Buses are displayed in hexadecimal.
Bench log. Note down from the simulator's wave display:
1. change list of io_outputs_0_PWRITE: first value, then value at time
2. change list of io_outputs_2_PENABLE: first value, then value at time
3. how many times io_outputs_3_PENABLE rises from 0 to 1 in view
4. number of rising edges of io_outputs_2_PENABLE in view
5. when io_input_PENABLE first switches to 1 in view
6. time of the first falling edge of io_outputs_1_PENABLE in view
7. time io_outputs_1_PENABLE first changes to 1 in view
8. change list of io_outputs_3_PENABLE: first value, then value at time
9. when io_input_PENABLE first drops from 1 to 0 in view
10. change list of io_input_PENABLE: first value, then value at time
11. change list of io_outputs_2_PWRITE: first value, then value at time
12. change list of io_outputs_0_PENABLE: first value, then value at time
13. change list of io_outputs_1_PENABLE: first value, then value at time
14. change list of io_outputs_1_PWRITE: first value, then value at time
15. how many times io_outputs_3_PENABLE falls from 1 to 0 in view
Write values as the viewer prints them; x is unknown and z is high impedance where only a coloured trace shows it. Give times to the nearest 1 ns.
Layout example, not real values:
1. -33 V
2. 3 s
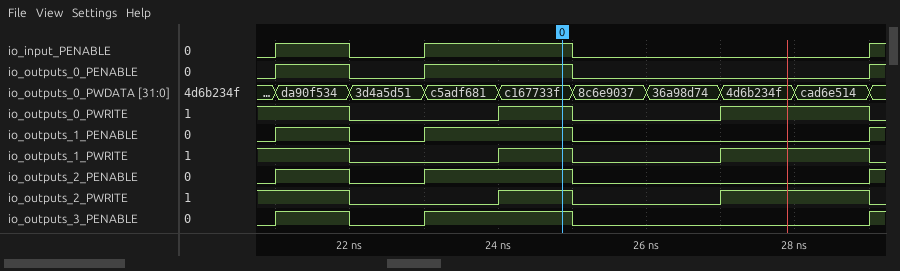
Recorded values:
1. 1, 0 at 22 ns, 1 at 24 ns, 0 at 25 ns, 1 at 27 ns, 0 at 29 ns
2. 0, 1 at 21 ns, 0 at 22 ns, 1 at 23 ns, 0 at 25 ns, 1 at 29 ns
3. 3
4. 3
5. 21 ns
6. 22 ns
7. 21 ns
8. 0, 1 at 21 ns, 0 at 22 ns, 1 at 23 ns, 0 at 25 ns, 1 at 29 ns
9. 22 ns
10. 0, 1 at 21 ns, 0 at 22 ns, 1 at 23 ns, 0 at 25 ns, 1 at 29 ns
11. 1, 0 at 22 ns, 1 at 24 ns, 0 at 25 ns, 1 at 27 ns, 0 at 29 ns
12. 0, 1 at 21 ns, 0 at 22 ns, 1 at 23 ns, 0 at 25 ns, 1 at 29 ns
13. 0, 1 at 21 ns, 0 at 22 ns, 1 at 23 ns, 0 at 25 ns, 1 at 29 ns
14. 1, 0 at 22 ns, 1 at 24 ns, 0 at 25 ns, 1 at 27 ns, 0 at 29 ns
15. 2
